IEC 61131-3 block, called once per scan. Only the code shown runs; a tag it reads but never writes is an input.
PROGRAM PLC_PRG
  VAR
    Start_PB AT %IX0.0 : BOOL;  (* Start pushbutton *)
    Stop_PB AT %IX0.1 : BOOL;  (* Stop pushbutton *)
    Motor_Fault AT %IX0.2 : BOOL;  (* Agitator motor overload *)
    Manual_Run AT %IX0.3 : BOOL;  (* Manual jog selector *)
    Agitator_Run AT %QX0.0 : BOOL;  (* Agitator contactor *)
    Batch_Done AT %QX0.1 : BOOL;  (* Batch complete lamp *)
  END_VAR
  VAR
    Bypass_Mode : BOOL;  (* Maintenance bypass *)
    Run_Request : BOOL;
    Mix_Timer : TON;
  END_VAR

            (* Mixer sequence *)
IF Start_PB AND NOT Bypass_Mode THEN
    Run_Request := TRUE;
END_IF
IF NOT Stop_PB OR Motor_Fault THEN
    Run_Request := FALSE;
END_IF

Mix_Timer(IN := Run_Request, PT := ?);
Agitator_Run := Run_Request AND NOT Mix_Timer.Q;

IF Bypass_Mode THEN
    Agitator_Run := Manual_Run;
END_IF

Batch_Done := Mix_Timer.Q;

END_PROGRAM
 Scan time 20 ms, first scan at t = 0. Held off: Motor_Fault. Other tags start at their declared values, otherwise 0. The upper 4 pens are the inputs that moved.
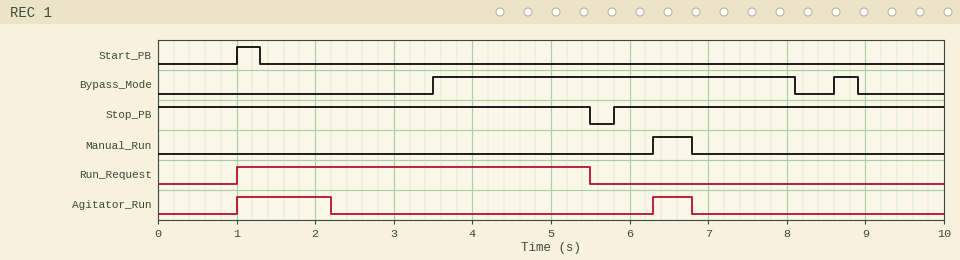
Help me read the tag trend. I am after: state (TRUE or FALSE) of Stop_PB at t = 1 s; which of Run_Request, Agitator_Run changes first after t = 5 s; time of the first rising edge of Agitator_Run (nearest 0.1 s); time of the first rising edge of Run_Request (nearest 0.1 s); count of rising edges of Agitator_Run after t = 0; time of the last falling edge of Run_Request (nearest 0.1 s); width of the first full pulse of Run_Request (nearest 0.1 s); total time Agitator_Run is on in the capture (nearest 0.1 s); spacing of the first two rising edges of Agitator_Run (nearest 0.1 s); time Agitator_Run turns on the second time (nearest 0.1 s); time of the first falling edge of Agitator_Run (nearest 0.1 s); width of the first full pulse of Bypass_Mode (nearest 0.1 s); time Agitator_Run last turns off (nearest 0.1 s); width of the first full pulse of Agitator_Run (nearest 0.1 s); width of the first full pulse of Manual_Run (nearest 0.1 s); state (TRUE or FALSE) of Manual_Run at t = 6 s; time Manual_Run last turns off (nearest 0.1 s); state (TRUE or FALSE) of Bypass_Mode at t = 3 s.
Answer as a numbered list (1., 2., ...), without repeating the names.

1. TRUE
2. Run_Request
3. 1.0 s
4. 1.0 s
5. 2
6. 5.5 s
7. 4.5 s
8. 1.7 s
9. 5.3 s
10. 6.3 s
11. 2.2 s
12. 4.6 s
13. 6.8 s
14. 1.2 s
15. 0.5 s
16. FALSE
17. 6.8 s
18. FALSE
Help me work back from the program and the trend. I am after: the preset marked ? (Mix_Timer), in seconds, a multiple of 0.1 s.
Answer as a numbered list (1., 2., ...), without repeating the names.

1. 1.2 s
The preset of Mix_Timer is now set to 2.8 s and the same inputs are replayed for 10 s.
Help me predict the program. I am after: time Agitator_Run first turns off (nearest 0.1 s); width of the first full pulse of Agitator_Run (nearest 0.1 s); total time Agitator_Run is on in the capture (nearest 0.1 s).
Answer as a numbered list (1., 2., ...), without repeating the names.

1. 3.5 s
2. 2.5 s
3. 3.0 s
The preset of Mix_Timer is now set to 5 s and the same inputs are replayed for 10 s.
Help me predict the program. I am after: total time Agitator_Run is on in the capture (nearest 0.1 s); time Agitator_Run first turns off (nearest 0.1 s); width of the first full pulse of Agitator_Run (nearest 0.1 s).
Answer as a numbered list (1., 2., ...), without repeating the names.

1. 3.0 s
2. 3.5 s
3. 2.5 s
